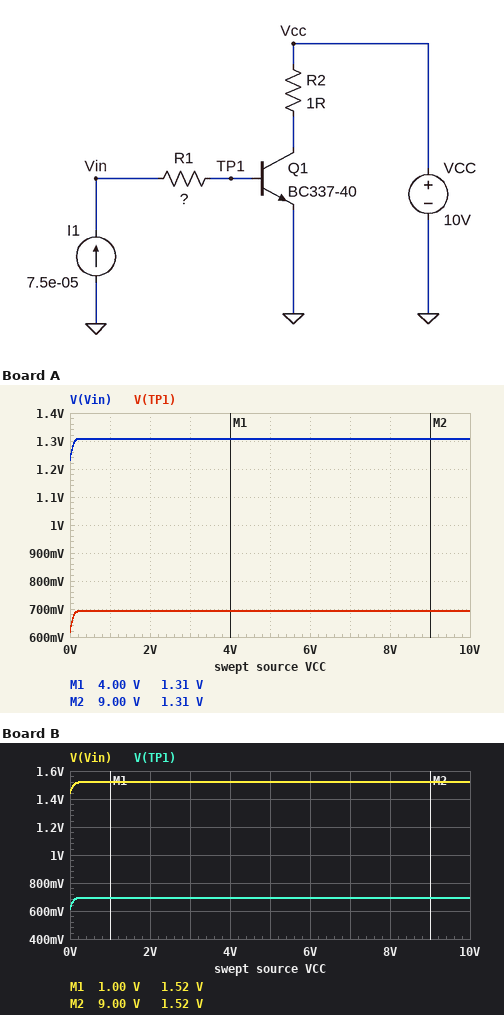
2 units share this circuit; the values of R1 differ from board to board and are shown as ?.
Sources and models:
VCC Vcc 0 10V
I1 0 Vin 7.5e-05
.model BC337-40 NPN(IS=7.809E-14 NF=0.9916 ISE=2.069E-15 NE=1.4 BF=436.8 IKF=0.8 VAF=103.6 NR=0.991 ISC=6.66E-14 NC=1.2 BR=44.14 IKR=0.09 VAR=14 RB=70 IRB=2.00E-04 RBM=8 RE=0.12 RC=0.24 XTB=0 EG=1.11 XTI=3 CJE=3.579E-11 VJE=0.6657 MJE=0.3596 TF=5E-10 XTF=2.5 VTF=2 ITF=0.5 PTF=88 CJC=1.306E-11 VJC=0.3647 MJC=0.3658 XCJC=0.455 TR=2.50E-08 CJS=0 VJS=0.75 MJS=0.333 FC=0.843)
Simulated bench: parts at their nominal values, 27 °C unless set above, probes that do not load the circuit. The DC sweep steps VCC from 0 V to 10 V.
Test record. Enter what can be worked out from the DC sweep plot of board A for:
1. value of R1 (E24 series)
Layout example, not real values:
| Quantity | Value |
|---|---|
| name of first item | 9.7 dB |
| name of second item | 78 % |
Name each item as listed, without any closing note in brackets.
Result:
| Quantity | Value |
|---|---|
| value of R1 | 8.2 kΩ |
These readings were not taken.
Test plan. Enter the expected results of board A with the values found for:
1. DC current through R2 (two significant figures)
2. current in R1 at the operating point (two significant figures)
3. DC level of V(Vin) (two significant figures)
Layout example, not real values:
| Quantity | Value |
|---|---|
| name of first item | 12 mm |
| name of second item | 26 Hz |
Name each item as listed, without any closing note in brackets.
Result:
| Quantity | Value |
|---|---|
| DC current through R2 | 33 mA |
| current in R1 at the operating point | 75 µA |
| DC level of V(Vin) | 1.3 V |
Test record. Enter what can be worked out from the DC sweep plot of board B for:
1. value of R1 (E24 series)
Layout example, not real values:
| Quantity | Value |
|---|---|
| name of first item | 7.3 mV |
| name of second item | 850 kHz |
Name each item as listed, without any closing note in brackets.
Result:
| Quantity | Value |
|---|---|
| value of R1 | 11 kΩ |
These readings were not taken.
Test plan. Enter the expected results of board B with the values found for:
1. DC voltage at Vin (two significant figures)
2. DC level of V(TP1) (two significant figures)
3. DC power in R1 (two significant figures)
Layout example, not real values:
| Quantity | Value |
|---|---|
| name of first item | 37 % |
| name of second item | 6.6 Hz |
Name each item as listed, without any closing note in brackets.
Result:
| Quantity | Value |
|---|---|
| DC voltage at Vin | 1.5 V |
| DC level of V(TP1) | 690 mV |
| DC power in R1 | 62 µW |
